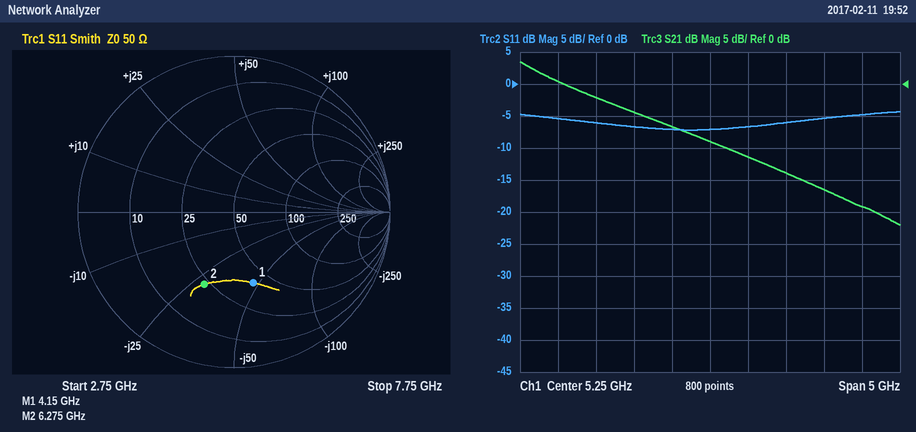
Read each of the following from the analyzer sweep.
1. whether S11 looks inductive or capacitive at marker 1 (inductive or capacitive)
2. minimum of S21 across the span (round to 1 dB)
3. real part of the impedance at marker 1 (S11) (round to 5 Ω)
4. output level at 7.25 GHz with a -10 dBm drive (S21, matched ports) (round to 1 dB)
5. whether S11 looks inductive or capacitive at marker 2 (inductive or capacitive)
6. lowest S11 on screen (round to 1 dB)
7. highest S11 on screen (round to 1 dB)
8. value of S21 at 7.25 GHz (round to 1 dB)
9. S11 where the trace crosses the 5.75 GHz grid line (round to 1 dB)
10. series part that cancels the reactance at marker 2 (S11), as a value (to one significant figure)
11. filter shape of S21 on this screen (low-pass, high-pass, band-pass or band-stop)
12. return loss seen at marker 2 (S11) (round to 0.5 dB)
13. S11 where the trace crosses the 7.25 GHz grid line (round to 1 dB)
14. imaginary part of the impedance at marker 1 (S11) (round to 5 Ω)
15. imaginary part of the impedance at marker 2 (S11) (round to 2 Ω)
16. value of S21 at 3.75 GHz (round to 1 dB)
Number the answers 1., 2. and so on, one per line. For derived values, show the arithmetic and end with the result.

1. capacitive
2. -22 dB
3. 40 Ω
4. -10 dBm + (-19 dB) = -29 dBm
5. capacitive
6. -7 dB
7. -4 dB
8. -19 dB
9. -7 dB
10. L = 28 Ω/(2π × 6.275 GHz) ≈ 710 pH, so 700 pH to one significant figure
11. low-pass
12. 6.0 dB
13. -5 dB
14. -45 Ω
15. -28 Ω
16. -2 dB
